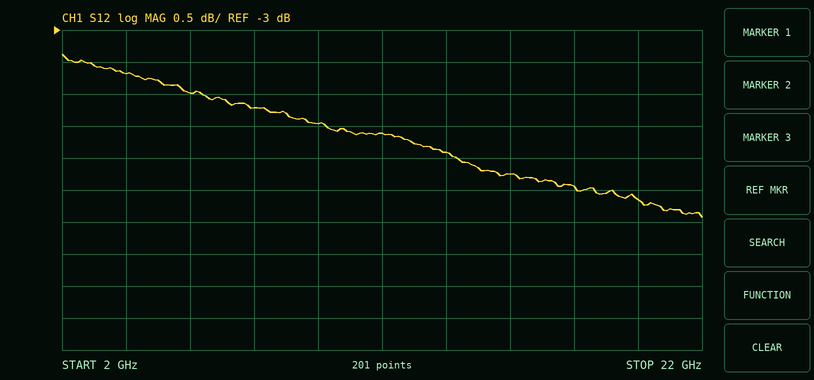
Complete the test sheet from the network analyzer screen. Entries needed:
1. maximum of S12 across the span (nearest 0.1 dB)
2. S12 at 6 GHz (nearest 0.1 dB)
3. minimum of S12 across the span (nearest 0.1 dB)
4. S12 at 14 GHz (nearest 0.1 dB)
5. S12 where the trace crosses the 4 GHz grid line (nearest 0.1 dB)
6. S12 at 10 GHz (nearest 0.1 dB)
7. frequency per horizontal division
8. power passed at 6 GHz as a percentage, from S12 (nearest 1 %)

-3.4 dB
-4.0 dB
-5.9 dB
-4.9 dB
-3.7 dB
-4.5 dB
2 GHz
40 %
